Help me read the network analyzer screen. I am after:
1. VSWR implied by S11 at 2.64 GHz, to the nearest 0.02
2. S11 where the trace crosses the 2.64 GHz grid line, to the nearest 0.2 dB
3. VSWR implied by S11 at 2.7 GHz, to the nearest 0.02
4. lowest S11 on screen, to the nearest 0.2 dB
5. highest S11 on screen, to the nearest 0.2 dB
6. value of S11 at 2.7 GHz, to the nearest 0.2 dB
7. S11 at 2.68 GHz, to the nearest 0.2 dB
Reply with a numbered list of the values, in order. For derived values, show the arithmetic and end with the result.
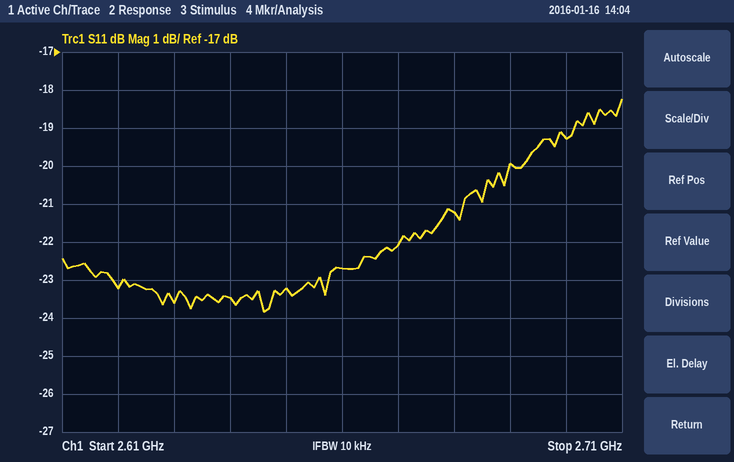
1. |Γ| = 10^(-23.4/20) = 0.0676; VSWR = (1 + 0.0676)/(1 − 0.0676) ≈ 1.15, so 1.14 to the nearest 0.02
2. -23.4 dB
3. |Γ| = 10^(-19.2/20) = 0.1096; VSWR = (1 + 0.1096)/(1 − 0.1096) ≈ 1.25, so 1.24 to the nearest 0.02
4. -23.8 dB
5. -18.2 dB
6. -19.2 dB
7. -21.2 dB
